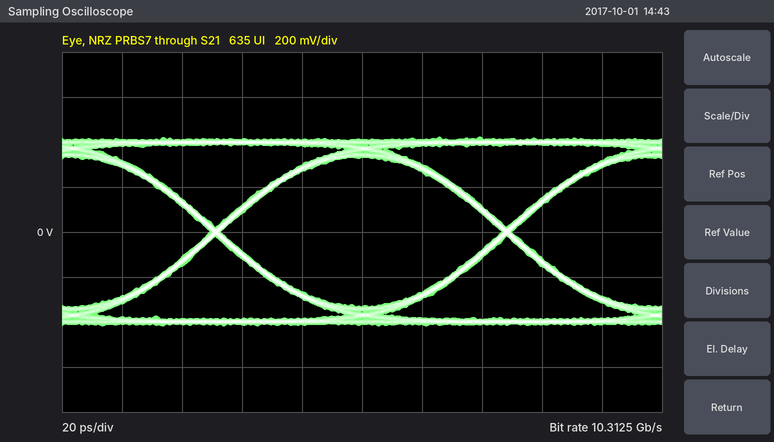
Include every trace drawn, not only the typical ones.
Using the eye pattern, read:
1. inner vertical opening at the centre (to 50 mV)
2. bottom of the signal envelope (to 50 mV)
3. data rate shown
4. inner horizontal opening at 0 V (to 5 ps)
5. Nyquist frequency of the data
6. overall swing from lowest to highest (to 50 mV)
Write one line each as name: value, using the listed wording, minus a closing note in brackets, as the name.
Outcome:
inner vertical opening at the centre: 650 mV
bottom of the signal envelope: -400 mV
data rate shown: 10.3125 Gb/s
inner horizontal opening at 0 V: 95 ps
Nyquist frequency of the data: 5.15625 GHz
overall swing from lowest to highest: 850 mV
